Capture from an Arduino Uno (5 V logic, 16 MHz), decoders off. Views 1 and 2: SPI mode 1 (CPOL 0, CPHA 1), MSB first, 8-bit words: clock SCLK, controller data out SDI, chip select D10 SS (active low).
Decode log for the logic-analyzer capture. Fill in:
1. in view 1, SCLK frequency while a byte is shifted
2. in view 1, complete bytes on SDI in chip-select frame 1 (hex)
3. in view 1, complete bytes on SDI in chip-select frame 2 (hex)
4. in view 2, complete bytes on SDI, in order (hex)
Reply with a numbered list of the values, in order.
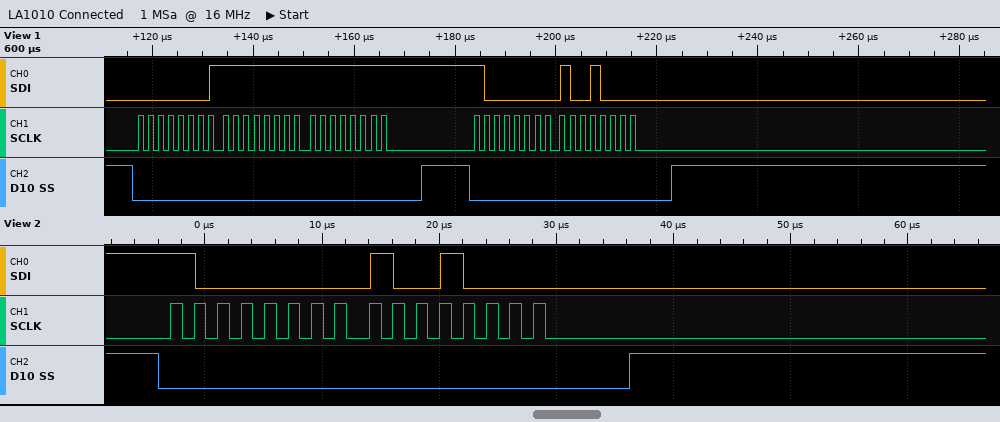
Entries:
1. 500 kHz
2. 0x01 0xFF 0xFF
3. 0x80 0x90
4. 80 90
